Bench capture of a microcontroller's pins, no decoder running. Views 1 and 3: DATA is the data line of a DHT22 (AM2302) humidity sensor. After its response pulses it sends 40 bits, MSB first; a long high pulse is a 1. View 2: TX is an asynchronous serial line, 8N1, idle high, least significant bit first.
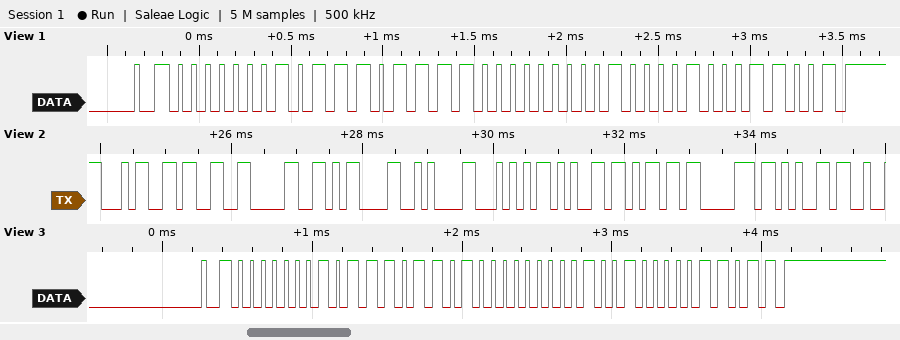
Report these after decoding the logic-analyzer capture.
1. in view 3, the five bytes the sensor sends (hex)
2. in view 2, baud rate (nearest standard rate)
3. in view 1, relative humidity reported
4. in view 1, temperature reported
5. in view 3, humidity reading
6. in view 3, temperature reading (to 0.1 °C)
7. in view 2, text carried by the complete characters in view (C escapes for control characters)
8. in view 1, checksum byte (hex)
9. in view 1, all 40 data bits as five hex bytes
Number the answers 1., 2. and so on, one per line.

1. 01 76 80 24 1B
2. 9600 baud
3. 37.5 %
4. -3.3 °C
5. 37.4 %
6. -3.6 °C
7. "430\r\nTempe"
8. 0x19
9. 01 77 80 21 19
